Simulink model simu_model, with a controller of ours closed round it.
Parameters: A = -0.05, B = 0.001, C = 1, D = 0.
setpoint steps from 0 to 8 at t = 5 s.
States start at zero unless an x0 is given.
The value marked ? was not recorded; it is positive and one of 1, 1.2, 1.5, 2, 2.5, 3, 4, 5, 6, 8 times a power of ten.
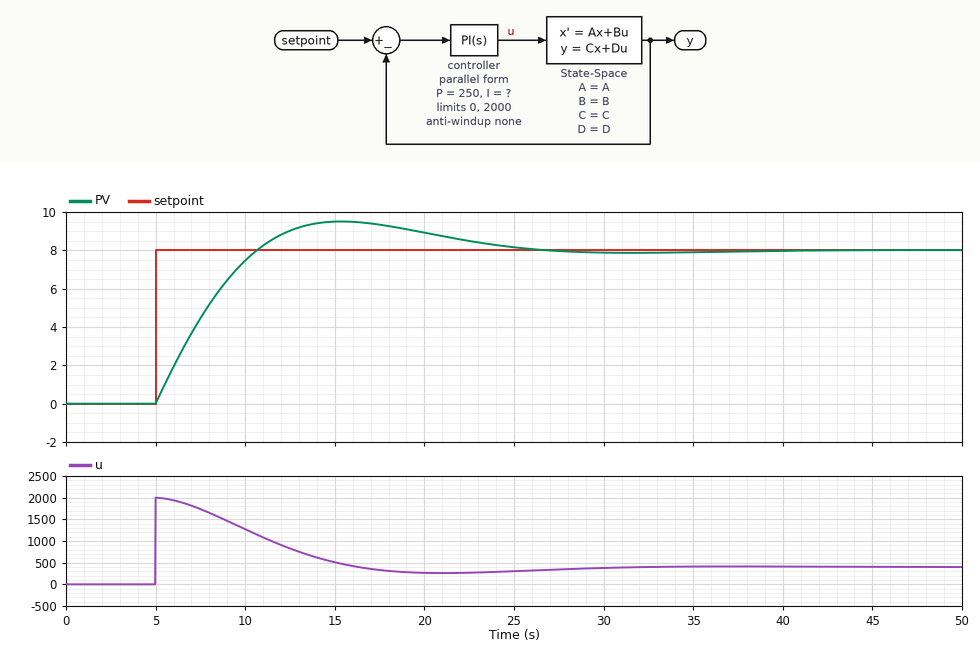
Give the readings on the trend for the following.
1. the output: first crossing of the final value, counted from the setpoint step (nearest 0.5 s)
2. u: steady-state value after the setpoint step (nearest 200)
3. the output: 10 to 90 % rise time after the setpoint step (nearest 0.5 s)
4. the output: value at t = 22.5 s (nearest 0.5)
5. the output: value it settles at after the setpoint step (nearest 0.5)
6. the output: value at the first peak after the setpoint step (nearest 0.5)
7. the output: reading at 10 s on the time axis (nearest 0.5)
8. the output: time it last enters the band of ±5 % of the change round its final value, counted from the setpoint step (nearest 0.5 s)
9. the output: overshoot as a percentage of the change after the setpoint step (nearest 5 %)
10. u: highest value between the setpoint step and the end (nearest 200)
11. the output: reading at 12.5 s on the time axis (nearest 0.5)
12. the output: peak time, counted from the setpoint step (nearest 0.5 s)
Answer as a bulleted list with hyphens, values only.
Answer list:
- 5.5 s
- 400
- 4.5 s
- 8.5
- 8.0
- 9.5
- 7.5
- 18.0 s
- 20 %
- 2000
- 9.0
- 10.5 s
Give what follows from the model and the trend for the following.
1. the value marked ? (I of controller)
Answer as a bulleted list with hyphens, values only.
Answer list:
- 60
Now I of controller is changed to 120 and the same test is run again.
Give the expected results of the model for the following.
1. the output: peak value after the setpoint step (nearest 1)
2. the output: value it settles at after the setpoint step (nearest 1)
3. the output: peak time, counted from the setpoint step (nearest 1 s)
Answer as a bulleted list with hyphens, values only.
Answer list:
- 11
- 8
- 8 s
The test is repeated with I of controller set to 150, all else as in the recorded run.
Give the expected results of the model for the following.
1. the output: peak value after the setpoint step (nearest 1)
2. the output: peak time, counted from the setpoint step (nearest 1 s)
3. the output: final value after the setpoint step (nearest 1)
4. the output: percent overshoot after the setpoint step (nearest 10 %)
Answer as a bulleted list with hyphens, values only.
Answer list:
- 11
- 8 s
- 8
- 40 %
